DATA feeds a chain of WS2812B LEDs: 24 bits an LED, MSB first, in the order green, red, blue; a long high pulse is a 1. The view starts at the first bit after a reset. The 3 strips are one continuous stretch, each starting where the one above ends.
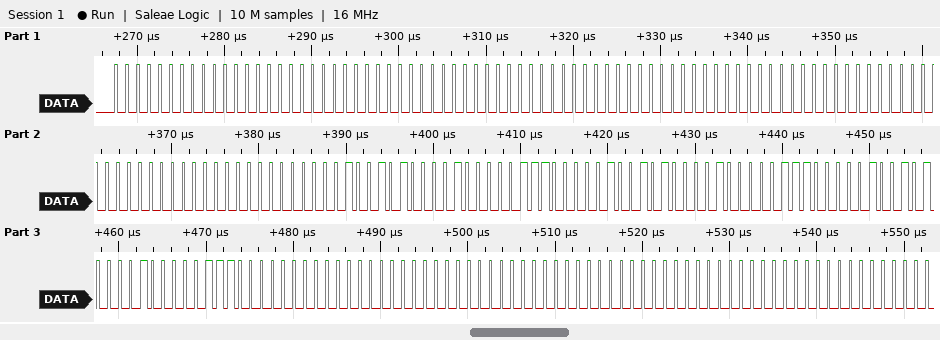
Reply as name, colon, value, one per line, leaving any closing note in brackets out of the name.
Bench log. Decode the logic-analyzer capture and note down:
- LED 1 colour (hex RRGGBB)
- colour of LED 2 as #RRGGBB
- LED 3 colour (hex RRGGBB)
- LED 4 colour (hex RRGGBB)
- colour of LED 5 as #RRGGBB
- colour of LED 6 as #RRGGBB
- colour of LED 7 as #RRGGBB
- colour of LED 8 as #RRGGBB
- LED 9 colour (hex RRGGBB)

LED 1 colour: #000000
colour of LED 2 as #RRGGBB: #000000
LED 3 colour: #000000
LED 4 colour: #000000
colour of LED 5 as #RRGGBB: #082538
colour of LED 6 as #RRGGBB: #082538
colour of LED 7 as #RRGGBB: #082538
colour of LED 8 as #RRGGBB: #000000
LED 9 colour: #000000
